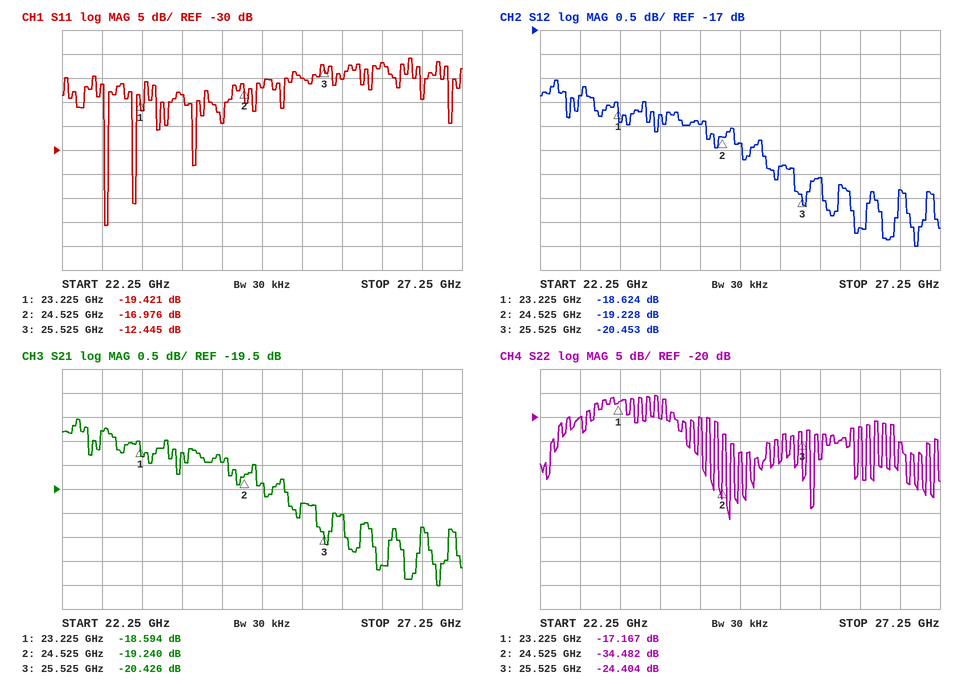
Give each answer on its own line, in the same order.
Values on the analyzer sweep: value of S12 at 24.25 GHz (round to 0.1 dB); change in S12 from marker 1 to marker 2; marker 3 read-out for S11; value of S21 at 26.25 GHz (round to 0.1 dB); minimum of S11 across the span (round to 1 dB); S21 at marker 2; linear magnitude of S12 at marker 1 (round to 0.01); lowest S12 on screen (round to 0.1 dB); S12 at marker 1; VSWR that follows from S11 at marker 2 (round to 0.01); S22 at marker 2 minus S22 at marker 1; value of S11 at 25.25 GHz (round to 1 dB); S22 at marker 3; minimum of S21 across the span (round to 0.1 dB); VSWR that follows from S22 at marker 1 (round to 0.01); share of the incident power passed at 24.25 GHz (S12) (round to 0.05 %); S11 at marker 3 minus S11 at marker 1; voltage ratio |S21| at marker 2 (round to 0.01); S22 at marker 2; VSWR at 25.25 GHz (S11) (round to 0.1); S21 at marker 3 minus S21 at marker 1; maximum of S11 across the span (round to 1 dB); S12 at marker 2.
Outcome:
-19.0 dB
-0.604 dB
-12.445 dB
-21.1 dB
-46 dB
-19.240 dB
0.12
-21.5 dB
-18.624 dB
1.33
-17.315 dB
-15 dB
-24.404 dB
-21.5 dB
1.32
1.25 %
6.976 dB
0.11
-34.482 dB
1.4
-1.832 dB
-11 dB
-19.228 dB
